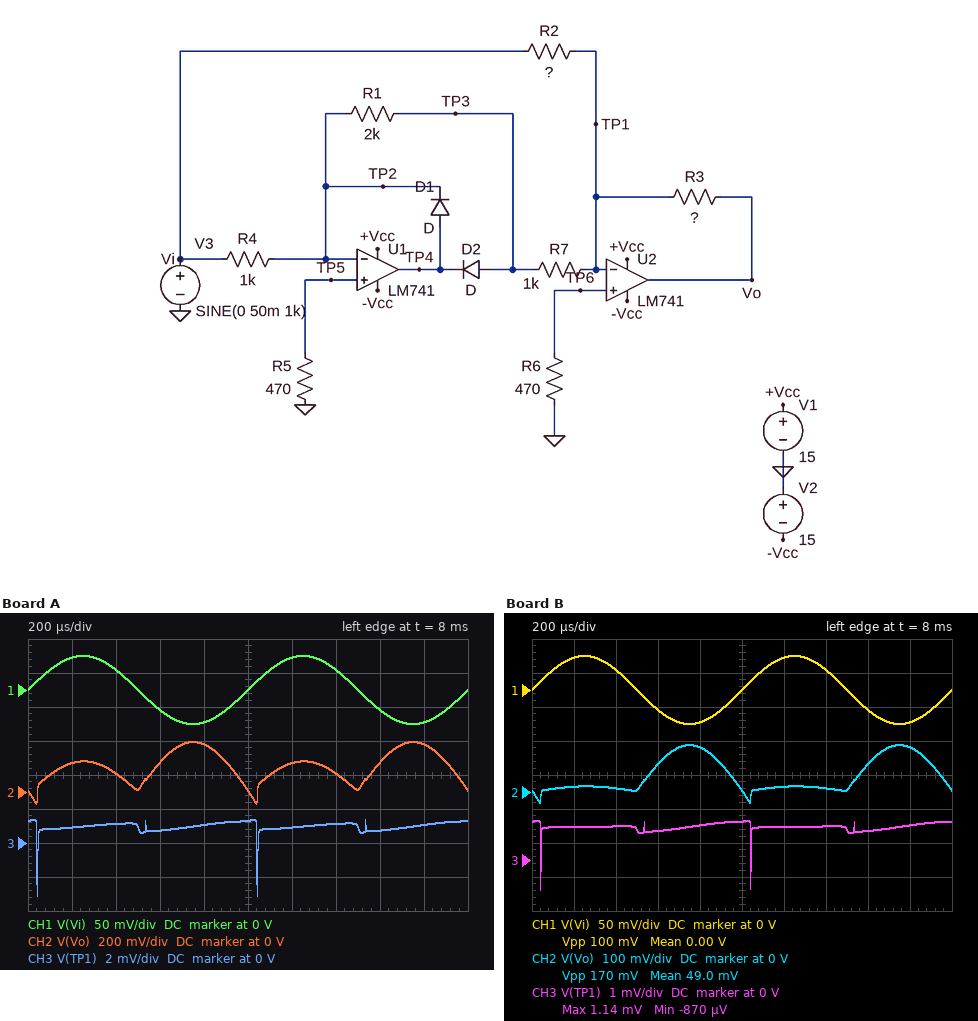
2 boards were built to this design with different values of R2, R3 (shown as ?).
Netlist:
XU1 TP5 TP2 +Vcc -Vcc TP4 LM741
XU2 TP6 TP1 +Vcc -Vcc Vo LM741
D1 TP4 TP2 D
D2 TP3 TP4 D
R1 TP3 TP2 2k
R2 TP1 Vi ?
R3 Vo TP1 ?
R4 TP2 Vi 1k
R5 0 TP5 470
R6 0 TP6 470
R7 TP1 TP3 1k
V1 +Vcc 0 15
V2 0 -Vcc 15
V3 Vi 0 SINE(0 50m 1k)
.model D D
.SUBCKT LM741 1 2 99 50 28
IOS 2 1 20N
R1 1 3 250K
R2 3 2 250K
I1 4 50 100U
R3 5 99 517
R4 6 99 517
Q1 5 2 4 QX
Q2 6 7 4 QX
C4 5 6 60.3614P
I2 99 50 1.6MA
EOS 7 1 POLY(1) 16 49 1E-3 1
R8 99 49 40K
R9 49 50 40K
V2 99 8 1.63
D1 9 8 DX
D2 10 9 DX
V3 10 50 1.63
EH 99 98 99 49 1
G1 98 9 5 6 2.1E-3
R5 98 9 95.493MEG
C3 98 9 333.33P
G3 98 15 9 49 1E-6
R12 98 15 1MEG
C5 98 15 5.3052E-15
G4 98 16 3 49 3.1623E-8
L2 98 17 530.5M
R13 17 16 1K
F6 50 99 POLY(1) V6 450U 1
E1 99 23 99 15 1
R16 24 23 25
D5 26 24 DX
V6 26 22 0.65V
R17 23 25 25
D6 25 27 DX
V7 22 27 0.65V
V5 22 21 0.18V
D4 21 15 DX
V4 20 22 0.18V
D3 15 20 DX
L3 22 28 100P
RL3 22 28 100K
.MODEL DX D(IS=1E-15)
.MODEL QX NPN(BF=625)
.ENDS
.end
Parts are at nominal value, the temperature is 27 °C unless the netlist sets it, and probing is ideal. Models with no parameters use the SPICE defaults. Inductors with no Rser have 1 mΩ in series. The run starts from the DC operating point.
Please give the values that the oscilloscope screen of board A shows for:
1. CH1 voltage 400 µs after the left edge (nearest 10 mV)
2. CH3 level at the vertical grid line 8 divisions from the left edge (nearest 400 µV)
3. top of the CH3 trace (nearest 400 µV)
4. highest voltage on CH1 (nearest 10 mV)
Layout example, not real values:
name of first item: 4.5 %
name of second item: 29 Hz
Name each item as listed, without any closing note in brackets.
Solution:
CH1 voltage 400 µs after the left edge: 30 mV
CH3 level at the vertical grid line 8 divisions from the left edge: 800 µV
top of the CH3 trace: 1.2 mV
highest voltage on CH1: 50 mV
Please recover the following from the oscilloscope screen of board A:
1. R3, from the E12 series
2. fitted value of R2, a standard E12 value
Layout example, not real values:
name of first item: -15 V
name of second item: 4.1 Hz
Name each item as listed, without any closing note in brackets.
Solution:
R3, from the E12 series: 4.7 kΩ
fitted value of R2, a standard E12 value: 820 Ω
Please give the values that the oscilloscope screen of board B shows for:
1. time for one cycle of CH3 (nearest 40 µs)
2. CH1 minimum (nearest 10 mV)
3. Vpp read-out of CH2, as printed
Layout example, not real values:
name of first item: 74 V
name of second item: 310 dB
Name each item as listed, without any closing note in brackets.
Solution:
time for one cycle of CH3: 1.00 ms
CH1 minimum: -50 mV
Vpp read-out of CH2, as printed: 170 mV
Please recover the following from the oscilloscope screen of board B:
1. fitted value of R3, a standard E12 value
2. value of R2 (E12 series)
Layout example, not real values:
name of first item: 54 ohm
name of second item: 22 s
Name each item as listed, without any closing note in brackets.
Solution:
fitted value of R3, a standard E12 value: 1.5 kΩ
value of R2: 560 Ω
